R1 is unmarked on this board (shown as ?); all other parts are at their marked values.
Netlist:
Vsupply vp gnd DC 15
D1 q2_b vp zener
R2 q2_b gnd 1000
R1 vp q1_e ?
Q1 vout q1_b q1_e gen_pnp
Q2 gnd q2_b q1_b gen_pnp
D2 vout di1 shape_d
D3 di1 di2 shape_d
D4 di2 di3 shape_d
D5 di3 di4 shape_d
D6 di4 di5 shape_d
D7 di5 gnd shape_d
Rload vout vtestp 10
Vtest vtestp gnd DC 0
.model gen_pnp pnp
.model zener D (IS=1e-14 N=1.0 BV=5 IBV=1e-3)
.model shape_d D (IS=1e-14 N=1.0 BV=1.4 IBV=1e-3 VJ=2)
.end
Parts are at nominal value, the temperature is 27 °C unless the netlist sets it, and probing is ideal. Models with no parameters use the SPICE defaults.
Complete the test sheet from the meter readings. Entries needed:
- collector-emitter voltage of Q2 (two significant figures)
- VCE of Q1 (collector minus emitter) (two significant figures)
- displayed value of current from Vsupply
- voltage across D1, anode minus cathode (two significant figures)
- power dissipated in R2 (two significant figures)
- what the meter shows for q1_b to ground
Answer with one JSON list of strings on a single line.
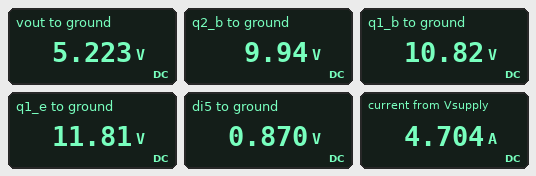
["-11 V", "-6.6 V", "4.704 A", "-5.1 V", "99 mW", "10.82 V"]
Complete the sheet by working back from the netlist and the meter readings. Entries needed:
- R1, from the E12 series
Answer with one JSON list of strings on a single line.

["0.68 Ω"]
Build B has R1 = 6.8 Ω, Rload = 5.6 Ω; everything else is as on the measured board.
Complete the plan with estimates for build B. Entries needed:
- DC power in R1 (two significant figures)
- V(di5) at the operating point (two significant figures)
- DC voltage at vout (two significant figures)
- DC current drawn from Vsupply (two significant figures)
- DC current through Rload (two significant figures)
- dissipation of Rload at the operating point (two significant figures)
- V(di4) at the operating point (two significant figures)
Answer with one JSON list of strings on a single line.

["1.6 W", "450 mV", "2.7 V", "500 mA", "480 mA", "1.3 W", "900 mV"]
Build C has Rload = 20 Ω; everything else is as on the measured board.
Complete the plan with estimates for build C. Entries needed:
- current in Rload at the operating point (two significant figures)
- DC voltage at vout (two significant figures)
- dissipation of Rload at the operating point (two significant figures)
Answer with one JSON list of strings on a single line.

["260 mA", "5.2 V", "1.4 W"]
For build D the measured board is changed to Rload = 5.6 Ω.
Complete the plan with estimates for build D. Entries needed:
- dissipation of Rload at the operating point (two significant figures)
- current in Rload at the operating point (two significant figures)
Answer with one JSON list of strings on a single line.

["4.8 W", "930 mA"]
